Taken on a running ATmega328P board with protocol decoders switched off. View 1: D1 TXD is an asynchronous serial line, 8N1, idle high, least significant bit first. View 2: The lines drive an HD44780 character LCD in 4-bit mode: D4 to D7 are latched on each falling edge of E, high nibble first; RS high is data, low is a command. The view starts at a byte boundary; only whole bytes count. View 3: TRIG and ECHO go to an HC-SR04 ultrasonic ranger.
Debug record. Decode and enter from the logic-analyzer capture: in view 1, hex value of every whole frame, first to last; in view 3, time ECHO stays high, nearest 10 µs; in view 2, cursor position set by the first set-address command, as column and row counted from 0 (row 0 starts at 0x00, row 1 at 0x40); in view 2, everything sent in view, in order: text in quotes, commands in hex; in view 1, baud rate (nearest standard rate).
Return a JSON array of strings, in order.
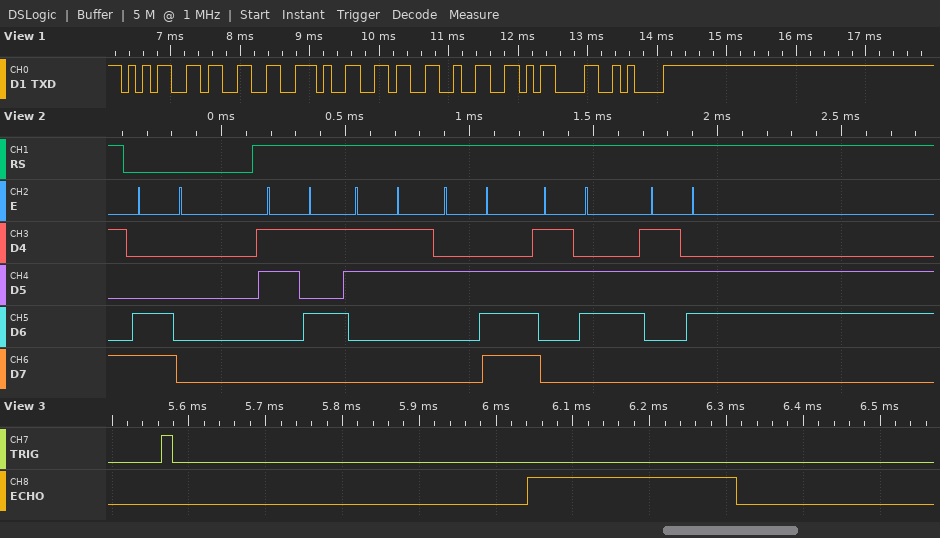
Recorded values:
["35 33 2E 36 32 0D 0A", "270 µs", "column 0, row 1", "0xC0 \"53.66\"", "9600 baud"]
